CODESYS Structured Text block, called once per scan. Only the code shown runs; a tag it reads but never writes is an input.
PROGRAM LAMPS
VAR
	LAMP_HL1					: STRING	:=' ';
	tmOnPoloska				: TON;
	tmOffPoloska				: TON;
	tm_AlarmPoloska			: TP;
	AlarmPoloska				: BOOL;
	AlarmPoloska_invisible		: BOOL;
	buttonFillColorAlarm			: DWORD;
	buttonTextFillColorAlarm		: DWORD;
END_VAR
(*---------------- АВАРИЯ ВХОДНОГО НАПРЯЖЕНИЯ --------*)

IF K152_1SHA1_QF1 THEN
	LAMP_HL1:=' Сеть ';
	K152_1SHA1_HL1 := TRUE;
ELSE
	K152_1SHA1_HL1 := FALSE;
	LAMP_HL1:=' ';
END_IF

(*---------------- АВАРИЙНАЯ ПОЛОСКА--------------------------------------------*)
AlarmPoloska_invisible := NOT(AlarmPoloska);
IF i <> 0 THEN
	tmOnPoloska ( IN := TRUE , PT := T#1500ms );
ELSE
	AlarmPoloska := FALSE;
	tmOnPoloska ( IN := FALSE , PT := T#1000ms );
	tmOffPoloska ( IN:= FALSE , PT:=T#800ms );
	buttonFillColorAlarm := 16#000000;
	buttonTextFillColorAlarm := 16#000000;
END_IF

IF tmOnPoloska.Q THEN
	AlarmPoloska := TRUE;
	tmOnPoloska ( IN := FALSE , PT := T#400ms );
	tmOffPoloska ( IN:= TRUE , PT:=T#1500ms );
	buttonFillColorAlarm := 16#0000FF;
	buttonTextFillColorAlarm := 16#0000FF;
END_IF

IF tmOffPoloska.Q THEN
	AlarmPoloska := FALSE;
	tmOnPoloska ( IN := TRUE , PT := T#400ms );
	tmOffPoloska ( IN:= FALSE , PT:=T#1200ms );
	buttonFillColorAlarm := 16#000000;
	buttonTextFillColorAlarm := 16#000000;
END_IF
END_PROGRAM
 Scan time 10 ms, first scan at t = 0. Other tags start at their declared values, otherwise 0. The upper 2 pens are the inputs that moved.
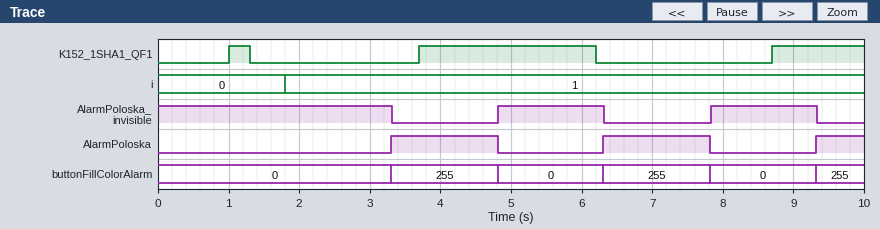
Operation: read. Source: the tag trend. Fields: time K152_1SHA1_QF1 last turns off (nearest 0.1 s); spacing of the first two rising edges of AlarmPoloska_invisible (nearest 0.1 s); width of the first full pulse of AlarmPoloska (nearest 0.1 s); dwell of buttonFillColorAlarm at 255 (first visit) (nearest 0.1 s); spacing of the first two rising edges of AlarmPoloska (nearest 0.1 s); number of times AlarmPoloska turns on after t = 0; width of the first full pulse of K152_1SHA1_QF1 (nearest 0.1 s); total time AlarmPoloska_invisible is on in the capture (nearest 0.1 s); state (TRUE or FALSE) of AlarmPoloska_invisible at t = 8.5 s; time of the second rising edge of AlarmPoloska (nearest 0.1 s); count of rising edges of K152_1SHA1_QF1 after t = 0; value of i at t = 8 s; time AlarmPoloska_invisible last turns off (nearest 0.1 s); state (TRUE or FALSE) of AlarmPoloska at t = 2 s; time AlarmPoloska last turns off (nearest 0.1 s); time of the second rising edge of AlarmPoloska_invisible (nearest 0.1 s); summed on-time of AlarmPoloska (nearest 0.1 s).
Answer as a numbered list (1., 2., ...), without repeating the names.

1. 6.2 s
2. 3.0 s
3. 1.5 s
4. 1.5 s
5. 3.0 s
6. 3
7. 0.3 s
8. 6.3 s
9. TRUE
10. 6.3 s
11. 3
12. 1
13. 9.3 s
14. FALSE
15. 7.8 s
16. 7.8 s
17. 3.7 s
